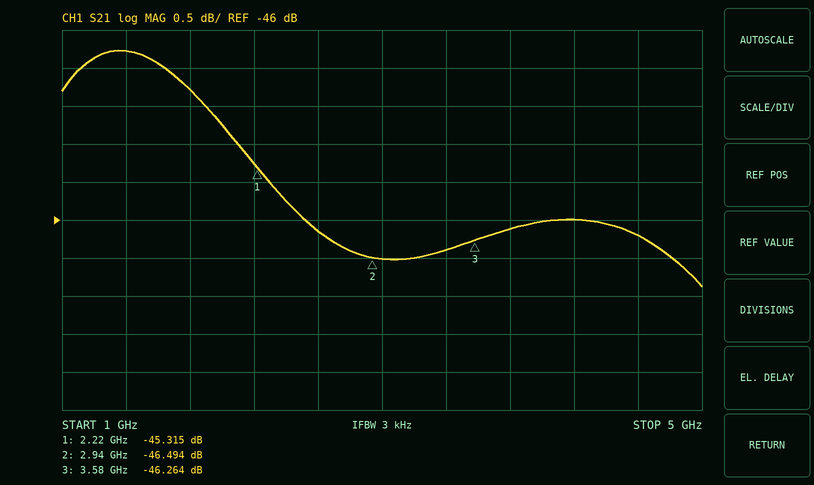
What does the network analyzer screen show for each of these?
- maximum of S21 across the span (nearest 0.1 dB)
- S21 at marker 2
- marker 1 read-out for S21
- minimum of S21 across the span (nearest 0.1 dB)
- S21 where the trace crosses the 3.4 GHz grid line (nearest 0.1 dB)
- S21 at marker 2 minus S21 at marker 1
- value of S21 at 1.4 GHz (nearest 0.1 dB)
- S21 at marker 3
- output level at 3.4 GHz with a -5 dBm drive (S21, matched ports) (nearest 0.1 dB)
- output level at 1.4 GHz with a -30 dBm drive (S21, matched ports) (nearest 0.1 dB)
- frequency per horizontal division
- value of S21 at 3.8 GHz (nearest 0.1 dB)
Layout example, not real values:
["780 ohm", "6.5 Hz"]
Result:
["-43.8 dB", "-46.494 dB", "-45.315 dB", "-46.9 dB", "-46.4 dB", "-1.179 dB", "-43.8 dB", "-46.264 dB", "-51.4 dBm", "-73.8 dBm", "400 MHz", "-46.1 dB"]
